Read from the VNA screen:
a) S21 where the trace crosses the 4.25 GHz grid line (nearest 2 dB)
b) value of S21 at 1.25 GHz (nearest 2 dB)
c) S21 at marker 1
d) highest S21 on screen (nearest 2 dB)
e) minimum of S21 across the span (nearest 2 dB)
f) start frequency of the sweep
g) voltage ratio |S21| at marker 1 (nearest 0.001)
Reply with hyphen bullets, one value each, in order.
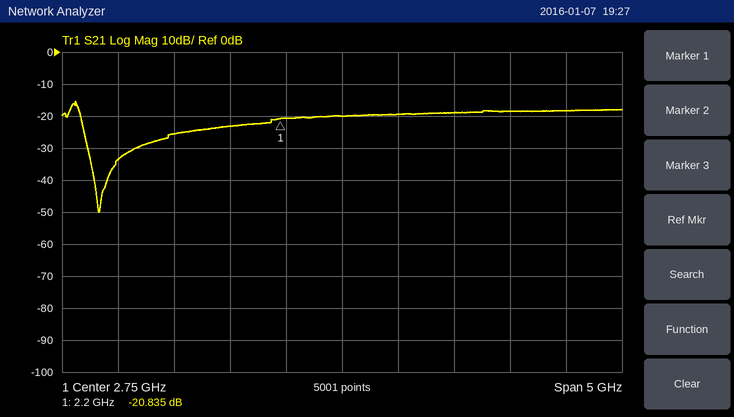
- -18 dB
- -26 dB
- -20.835 dB
- -16 dB
- -50 dB
- 250 MHz
- 0.091
